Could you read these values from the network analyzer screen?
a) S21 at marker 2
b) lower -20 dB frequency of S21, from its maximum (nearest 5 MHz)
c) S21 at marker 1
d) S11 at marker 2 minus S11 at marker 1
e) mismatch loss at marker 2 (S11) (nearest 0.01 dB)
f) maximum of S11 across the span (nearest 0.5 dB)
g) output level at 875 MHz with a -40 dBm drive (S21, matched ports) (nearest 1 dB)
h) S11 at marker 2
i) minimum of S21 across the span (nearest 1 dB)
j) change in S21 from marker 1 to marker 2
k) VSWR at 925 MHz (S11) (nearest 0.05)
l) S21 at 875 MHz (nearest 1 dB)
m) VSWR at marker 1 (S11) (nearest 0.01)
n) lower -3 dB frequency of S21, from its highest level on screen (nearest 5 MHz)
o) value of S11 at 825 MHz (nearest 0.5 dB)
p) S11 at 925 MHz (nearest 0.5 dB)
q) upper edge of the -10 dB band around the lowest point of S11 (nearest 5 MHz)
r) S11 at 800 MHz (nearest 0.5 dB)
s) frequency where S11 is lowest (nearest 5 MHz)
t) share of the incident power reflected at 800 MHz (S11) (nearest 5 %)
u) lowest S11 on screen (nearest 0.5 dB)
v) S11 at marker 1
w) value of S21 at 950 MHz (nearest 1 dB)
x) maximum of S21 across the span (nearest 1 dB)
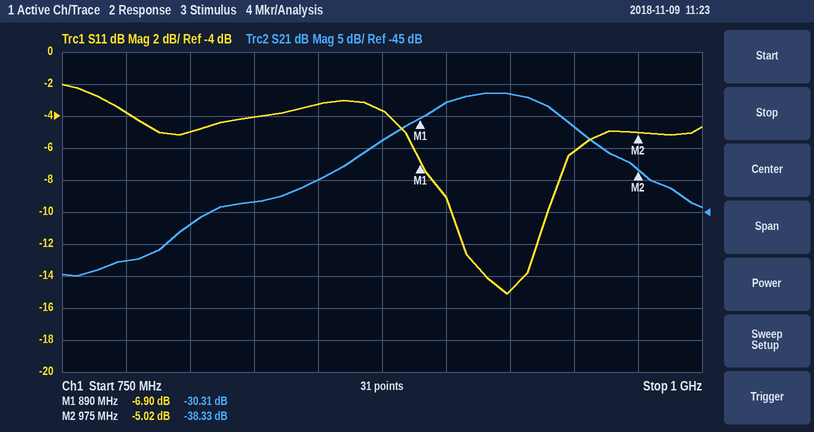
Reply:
-38.33 dB
800 MHz
-30.31 dB
1.88 dB
1.64 dB
-2.0 dB
-74 dBm
-5.02 dB
-55 dB
-8.02 dB
1.45
-34 dB
2.65
895 MHz
-4.0 dB
-15.0 dB
940 MHz
-5.0 dB
925 MHz
30 %
-15.0 dB
-6.90 dB
-32 dB
-26 dB
